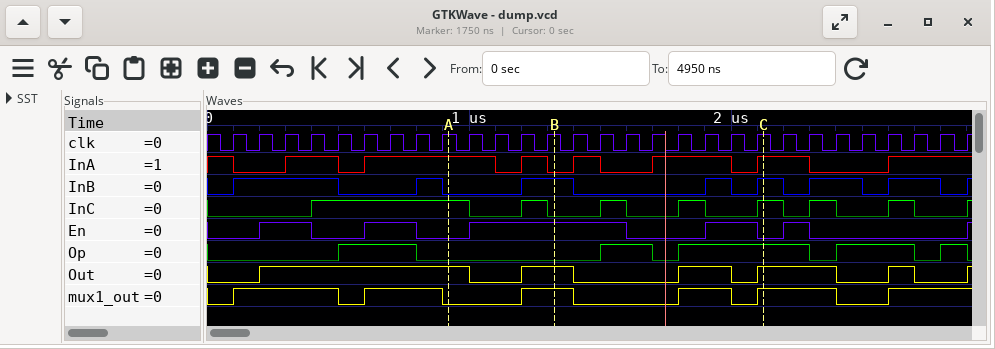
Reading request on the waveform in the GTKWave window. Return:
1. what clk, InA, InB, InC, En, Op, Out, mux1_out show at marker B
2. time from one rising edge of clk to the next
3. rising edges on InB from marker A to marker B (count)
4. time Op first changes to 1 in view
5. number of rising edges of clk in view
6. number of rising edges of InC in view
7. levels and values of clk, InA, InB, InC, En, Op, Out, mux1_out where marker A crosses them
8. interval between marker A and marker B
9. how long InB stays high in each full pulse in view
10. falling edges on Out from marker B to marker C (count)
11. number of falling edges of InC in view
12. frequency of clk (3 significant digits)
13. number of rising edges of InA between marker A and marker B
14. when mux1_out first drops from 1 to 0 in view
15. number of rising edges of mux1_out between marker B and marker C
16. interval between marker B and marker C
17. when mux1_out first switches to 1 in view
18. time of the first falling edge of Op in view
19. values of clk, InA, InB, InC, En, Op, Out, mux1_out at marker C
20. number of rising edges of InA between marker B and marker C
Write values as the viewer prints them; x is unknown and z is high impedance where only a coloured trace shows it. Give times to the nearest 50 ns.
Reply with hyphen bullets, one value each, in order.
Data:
- clk=1, InA=0, InB=1, InC=0, En=1, Op=0, Out=1, mux1_out=1
- 100 ns
- 1
- 500 ns
- 29
- 8
- clk=1, InA=1, InB=0, InC=1, En=0, Op=0, Out=1, mux1_out=0
- 400 ns
- 400 ns, 100 ns, 200 ns, 100 ns, 100 ns, 200 ns, 200 ns
- 2
- 7
- 10.0 MHz
- 1
- 500 ns
- 2
- 800 ns
- 100 ns
- 800 ns
- clk=1, InA=1, InB=1, InC=1, En=0, Op=1, Out=1, mux1_out=1
- 3
